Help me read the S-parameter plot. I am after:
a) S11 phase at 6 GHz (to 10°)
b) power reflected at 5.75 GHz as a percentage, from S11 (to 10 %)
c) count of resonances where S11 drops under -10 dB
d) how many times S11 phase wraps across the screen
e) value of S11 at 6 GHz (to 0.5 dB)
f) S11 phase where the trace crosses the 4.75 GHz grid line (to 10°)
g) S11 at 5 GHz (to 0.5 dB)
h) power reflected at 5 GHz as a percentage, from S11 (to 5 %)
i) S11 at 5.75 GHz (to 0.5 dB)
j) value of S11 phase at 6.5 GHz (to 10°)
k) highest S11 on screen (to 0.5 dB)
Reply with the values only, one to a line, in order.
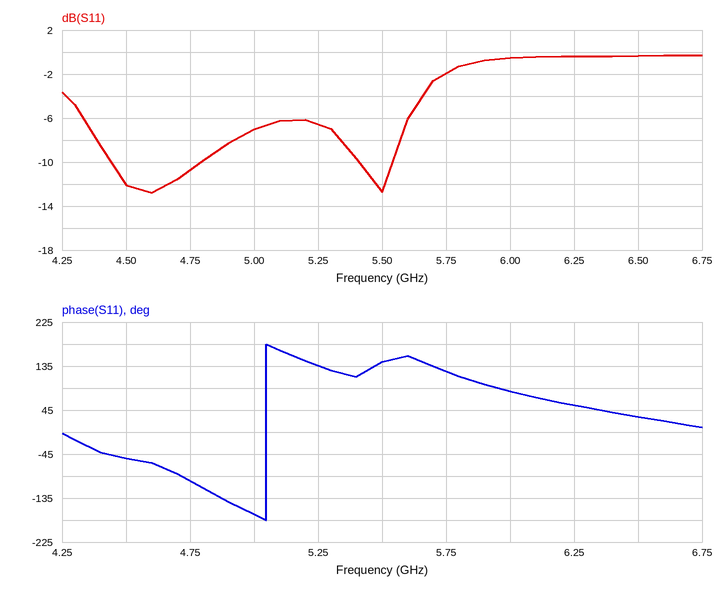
80°
60 %
2
1
-0.5 dB
-100°
-7.0 dB
20 %
-2.0 dB
30°
-0.5 dB
